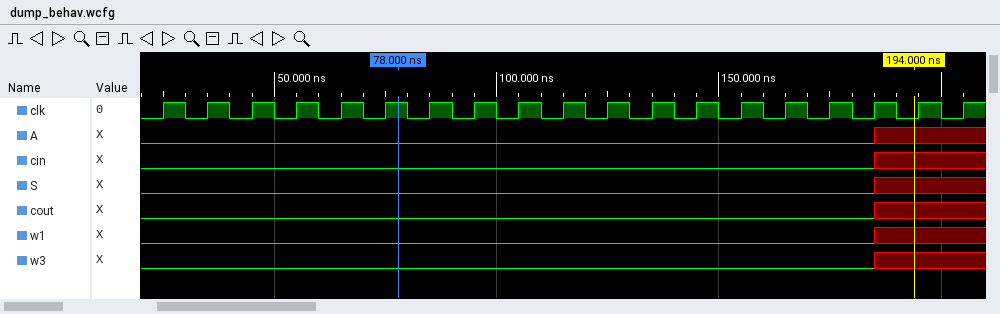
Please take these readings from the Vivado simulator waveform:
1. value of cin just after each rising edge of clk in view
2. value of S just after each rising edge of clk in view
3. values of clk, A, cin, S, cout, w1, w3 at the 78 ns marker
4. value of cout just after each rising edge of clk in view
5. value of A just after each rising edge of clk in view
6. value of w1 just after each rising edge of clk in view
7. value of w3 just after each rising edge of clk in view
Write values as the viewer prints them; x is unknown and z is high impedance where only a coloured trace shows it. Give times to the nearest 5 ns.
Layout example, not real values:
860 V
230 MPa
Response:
0 0 0 0 0 0 0 0 0 0 0 0 0 0 0 0 x x x
0 0 0 0 0 0 0 0 0 0 0 0 0 0 0 0 x x x
clk=1, A=0, cin=0, S=0, cout=0, w1=0, w3=0
0 0 0 0 0 0 0 0 0 0 0 0 0 0 0 0 x x x
0 0 0 0 0 0 0 0 0 0 0 0 0 0 0 0 x x x
0 0 0 0 0 0 0 0 0 0 0 0 0 0 0 0 x x x
0 0 0 0 0 0 0 0 0 0 0 0 0 0 0 0 x x x
